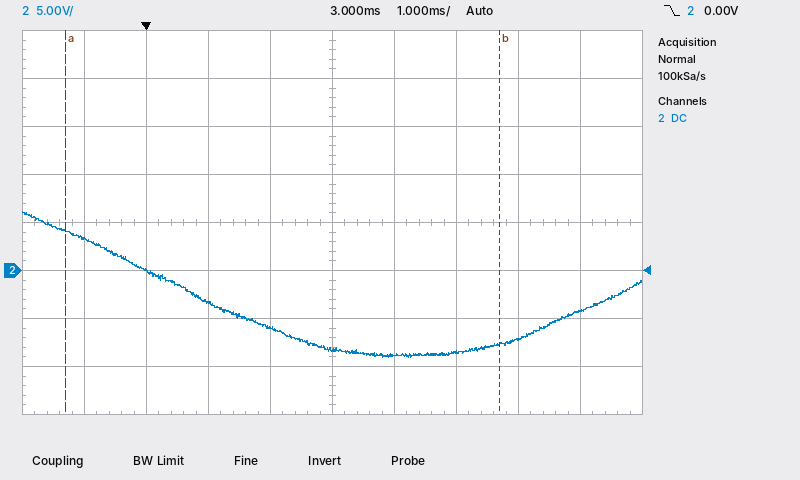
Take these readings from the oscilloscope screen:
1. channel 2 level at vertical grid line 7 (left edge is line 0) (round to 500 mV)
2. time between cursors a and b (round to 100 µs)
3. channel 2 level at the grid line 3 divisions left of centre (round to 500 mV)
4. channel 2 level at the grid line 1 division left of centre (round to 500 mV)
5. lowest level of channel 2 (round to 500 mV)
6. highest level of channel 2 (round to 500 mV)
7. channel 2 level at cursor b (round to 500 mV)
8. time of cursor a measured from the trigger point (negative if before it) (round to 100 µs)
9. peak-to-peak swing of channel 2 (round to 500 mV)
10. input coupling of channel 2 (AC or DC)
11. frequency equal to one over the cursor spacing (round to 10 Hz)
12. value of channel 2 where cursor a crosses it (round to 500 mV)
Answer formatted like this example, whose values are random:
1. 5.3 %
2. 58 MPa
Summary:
1. -8.5 V
2. 7.0 ms
3. 0.0 V
4. -6.0 V
5. -9.0 V
6. 6.0 V
7. -7.5 V
8. -1.3 ms
9. 15.0 V
10. DC
11. 140 Hz
12. 4.0 V
